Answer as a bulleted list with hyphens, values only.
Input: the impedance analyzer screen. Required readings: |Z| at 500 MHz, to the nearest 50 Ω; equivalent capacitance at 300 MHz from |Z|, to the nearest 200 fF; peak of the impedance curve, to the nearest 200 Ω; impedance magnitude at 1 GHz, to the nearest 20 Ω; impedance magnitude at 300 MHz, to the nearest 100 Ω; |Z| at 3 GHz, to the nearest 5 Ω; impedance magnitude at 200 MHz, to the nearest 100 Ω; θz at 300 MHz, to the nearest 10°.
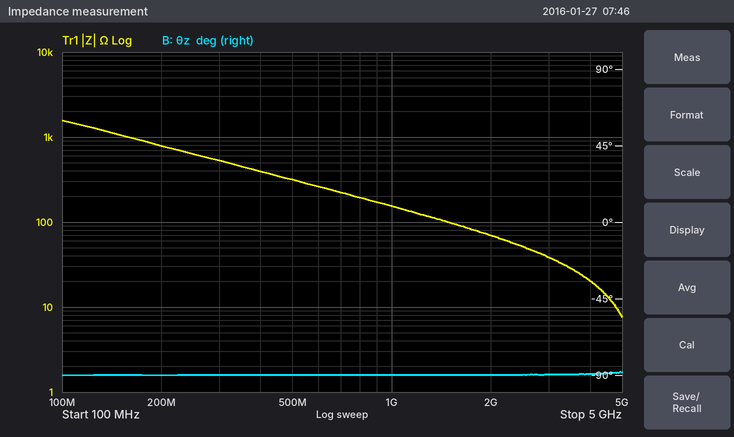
- 300 Ω
- 1.0 pF
- 1.6 kΩ
- 160 Ω
- 500 Ω
- 40 Ω
- 800 Ω
- -90°
